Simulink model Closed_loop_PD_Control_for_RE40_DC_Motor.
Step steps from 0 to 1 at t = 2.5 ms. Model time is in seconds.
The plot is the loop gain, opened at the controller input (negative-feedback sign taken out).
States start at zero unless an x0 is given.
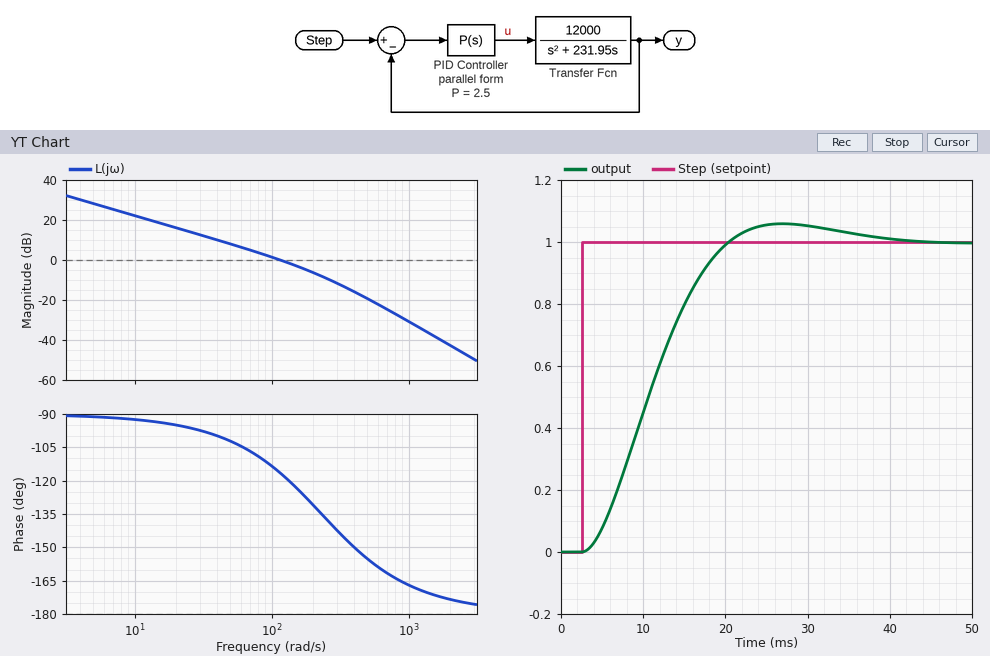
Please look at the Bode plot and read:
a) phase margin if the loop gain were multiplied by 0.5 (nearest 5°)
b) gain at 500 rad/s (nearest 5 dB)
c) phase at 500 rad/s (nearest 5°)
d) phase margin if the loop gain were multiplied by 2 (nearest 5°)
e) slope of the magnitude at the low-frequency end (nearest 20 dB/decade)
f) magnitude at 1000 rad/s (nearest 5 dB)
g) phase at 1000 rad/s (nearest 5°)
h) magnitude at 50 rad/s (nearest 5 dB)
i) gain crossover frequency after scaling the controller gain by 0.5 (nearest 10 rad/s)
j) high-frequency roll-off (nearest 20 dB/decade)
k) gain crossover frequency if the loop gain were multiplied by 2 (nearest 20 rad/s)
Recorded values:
75°
-20 dB
-155°
50°
-20 dB/decade
-30 dB
-165°
10 dB
60 rad/s
-40 dB/decade
200 rad/s
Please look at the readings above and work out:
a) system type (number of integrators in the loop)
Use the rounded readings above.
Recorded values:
1
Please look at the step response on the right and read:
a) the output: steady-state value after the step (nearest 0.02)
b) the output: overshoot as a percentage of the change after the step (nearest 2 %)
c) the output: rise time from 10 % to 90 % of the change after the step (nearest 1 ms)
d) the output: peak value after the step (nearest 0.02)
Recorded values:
1.00
6 %
12 ms
1.06
